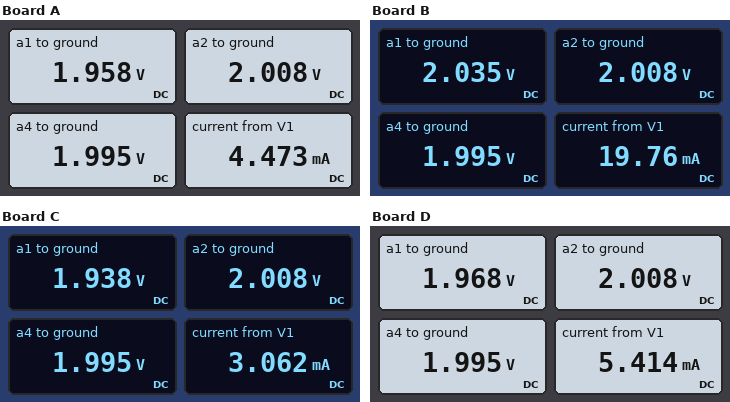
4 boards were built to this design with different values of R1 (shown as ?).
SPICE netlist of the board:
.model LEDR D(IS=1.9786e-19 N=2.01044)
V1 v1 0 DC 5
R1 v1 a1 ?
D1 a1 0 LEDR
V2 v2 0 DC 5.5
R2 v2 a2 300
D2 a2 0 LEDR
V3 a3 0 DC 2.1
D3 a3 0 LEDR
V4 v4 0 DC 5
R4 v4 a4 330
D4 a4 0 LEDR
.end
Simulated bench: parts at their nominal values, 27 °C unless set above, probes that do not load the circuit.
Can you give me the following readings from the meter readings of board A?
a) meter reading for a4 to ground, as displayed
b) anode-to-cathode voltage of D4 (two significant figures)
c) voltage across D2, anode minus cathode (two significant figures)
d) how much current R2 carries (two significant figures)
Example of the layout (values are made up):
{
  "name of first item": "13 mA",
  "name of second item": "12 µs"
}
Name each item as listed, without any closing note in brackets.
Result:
{
  "meter reading for a4 to ground, as displayed": "1.995 V",
  "anode-to-cathode voltage of D4": "2.0 V",
  "voltage across D2, anode minus cathode": "2.0 V",
  "how much current R2 carries": "12 mA"
}
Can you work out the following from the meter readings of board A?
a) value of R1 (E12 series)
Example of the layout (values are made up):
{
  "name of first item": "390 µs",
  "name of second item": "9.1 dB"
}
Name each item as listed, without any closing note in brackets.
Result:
{
  "value of R1": "680 Ω"
}
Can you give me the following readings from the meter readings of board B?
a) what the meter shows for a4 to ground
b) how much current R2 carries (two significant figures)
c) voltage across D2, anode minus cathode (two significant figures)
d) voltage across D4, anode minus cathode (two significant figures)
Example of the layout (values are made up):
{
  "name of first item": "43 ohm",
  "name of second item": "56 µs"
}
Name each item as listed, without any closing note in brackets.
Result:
{
  "what the meter shows for a4 to ground": "1.995 V",
  "how much current R2 carries": "12 mA",
  "voltage across D2, anode minus cathode": "2.0 V",
  "voltage across D4, anode minus cathode": "2.0 V"
}
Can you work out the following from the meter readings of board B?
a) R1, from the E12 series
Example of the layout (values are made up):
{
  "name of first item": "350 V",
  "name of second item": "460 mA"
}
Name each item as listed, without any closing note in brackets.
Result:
{
  "R1, from the E12 series": "150 Ω"
}
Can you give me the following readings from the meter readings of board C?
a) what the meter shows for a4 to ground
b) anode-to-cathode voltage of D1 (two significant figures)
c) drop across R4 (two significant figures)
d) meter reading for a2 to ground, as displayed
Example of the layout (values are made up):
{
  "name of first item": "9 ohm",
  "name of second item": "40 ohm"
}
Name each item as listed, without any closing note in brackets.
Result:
{
  "what the meter shows for a4 to ground": "1.995 V",
  "anode-to-cathode voltage of D1": "1.9 V",
  "drop across R4": "3.0 V",
  "meter reading for a2 to ground, as displayed": "2.008 V"
}
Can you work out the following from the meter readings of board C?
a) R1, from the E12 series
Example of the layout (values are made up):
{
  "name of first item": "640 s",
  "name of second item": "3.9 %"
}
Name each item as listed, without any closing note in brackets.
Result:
{
  "R1, from the E12 series": "1 kΩ"
}
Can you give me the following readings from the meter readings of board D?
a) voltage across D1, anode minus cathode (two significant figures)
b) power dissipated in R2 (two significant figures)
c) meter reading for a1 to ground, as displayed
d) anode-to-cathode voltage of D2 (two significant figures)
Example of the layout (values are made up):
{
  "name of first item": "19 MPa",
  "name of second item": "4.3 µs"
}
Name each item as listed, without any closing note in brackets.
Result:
{
  "voltage across D1, anode minus cathode": "2.0 V",
  "power dissipated in R2": "41 mW",
  "meter reading for a1 to ground, as displayed": "1.968 V",
  "anode-to-cathode voltage of D2": "2.0 V"
}
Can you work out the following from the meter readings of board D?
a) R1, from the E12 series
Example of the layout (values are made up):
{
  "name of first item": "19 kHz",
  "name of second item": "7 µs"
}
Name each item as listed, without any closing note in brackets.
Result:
{
  "R1, from the E12 series": "560 Ω"
}
